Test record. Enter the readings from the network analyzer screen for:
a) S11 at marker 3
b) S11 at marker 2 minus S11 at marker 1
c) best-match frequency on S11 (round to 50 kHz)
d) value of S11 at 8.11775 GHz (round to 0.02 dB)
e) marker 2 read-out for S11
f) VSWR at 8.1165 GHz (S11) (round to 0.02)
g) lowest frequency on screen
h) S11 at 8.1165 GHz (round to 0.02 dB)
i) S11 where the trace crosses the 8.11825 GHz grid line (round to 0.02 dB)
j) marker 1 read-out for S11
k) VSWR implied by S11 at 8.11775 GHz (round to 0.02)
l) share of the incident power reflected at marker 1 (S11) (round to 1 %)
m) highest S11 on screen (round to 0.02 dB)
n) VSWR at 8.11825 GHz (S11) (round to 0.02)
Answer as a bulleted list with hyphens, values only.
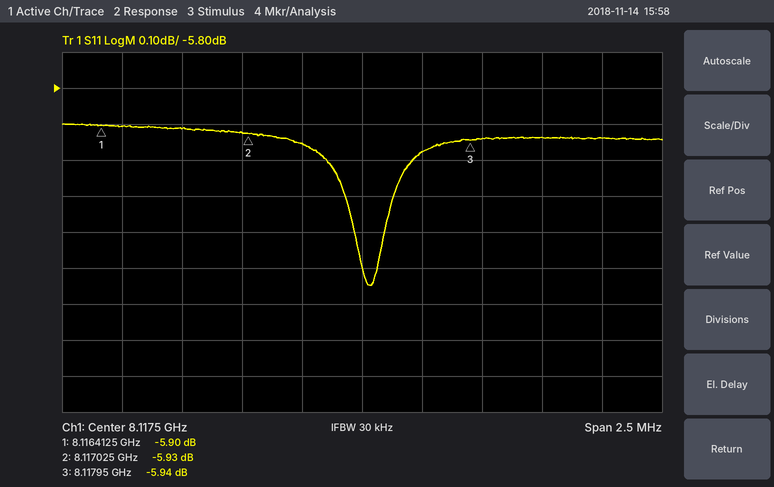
- -5.94 dB
- -0.03 dB
- 8.11755 GHz
- -5.98 dB
- -5.93 dB
- 3.06
- 8.11625 GHz
- -5.90 dB
- -5.94 dB
- -5.90 dB
- 3.02
- 26 %
- -5.90 dB
- 3.04
